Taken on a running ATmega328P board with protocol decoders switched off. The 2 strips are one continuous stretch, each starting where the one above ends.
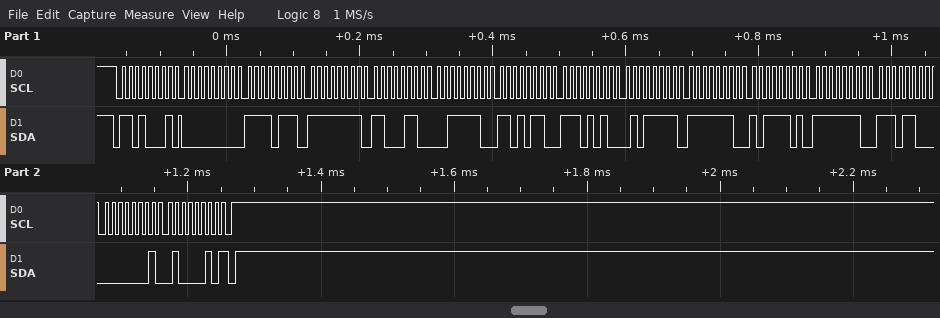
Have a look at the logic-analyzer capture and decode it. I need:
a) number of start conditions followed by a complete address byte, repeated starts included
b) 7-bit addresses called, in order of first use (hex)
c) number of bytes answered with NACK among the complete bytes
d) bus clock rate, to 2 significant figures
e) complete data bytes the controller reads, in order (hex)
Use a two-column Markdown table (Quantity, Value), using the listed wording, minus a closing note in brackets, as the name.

| Quantity | Value |
|---|---|
| number of start conditions followed by a complete address byte, repeated starts included | 1 |
| 7-bit addresses called, in order of first use | 0x68 |
| number of bytes answered with NACK among the complete bytes | 1 |
| bus clock rate, to 2 significant figures | 100 kHz |
| complete data bytes the controller reads, in order | 00 F7 FF C6 3E D6 EA 5F FE BD FE EC 01 42 |
